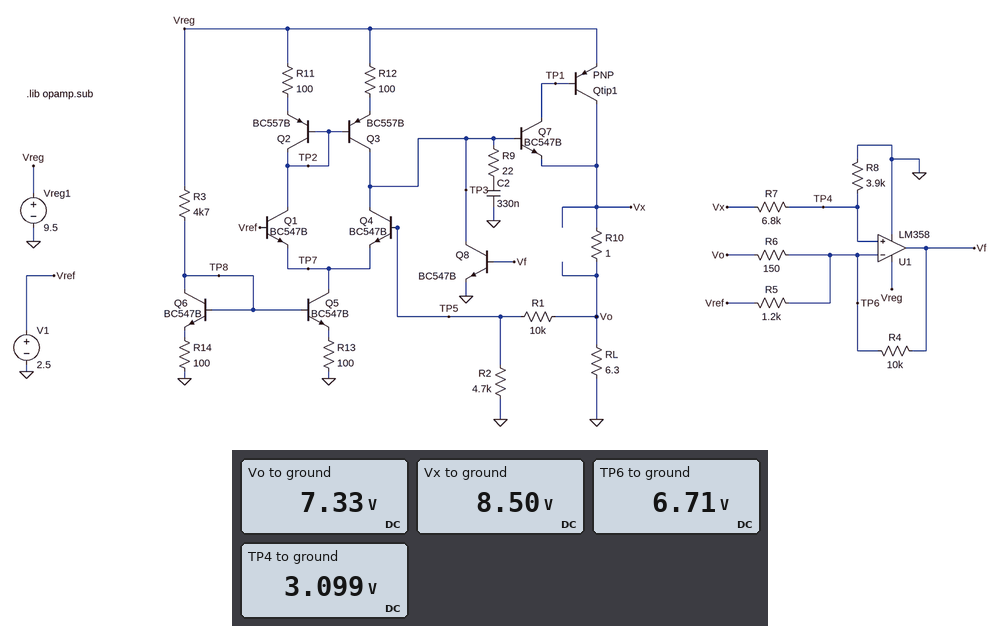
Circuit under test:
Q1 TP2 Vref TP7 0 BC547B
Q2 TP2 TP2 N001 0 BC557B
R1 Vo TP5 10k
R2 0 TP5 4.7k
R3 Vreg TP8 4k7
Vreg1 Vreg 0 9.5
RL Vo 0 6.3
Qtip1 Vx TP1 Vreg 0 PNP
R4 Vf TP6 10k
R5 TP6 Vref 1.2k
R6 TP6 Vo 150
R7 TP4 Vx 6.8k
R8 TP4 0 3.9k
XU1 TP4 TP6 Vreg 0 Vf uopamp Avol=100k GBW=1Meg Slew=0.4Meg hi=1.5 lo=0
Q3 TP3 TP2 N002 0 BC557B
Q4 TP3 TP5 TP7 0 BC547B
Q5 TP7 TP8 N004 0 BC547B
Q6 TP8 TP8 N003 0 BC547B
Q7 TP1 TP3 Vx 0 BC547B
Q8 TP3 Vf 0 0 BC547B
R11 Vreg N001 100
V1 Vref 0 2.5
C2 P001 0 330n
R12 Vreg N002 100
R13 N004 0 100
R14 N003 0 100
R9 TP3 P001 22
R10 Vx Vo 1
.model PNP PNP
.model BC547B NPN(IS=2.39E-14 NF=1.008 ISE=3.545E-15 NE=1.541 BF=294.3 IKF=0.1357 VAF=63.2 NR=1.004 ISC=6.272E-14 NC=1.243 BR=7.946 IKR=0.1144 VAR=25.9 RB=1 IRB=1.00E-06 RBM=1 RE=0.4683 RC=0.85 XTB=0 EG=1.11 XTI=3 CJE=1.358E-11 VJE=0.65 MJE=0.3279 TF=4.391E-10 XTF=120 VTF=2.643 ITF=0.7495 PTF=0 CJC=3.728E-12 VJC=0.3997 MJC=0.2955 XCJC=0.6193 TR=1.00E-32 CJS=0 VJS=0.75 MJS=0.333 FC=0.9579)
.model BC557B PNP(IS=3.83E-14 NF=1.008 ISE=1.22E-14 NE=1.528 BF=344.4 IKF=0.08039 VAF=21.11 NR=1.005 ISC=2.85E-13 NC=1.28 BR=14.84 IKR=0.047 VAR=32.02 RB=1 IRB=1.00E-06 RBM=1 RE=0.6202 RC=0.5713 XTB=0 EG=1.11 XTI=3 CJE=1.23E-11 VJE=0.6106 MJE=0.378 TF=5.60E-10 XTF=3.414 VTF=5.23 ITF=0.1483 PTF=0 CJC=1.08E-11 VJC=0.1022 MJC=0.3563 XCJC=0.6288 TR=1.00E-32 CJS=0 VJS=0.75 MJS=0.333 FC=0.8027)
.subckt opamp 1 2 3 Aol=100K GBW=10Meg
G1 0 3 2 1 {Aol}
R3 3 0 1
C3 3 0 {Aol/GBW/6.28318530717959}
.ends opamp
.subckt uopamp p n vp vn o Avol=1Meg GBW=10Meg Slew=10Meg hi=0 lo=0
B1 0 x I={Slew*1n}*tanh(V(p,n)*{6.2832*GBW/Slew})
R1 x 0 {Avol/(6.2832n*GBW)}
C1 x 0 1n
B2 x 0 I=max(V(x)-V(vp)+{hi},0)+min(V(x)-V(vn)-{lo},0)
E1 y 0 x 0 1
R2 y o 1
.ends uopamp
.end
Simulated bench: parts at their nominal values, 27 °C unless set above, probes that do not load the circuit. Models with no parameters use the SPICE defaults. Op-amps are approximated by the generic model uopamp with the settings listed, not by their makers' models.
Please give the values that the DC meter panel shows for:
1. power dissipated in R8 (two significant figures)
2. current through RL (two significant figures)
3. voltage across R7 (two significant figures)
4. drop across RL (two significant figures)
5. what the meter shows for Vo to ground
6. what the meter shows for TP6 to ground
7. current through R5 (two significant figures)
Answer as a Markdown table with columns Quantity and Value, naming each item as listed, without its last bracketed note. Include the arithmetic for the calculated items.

| Quantity | Value |
|---|---|
| power dissipated in R8 | (3.099 V)^2 / 3.9 kΩ = 2.5 mW |
| current through RL | (7.33 V) / 6.3 Ω = 1.2 A |
| voltage across R7 | 8.5 V - 3.099 V = 5.4 V |
| drop across RL | 7.33 V = 7.3 V |
| what the meter shows for Vo to ground | 7.33 V |
| what the meter shows for TP6 to ground | 6.71 V |
| current through R5 | (6.71 V - 2.5 V) / 1.2 kΩ = 3.5 mA |
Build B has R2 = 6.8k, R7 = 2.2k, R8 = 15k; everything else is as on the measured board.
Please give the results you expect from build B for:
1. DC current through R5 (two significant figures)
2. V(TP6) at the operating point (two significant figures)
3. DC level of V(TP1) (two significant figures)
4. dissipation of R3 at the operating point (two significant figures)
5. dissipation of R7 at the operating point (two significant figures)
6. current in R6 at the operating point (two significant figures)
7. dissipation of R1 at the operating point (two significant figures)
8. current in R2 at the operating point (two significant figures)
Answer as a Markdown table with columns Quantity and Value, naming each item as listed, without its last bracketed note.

| Quantity | Value |
|---|---|
| DC current through R5 | 300 µA |
| V(TP6) at the operating point | 2.1 V |
| DC level of V(TP1) | 8.6 V |
| dissipation of R3 at the operating point | 16 mW |
| dissipation of R7 at the operating point | 45 µW |
| current in R6 at the operating point | 150 µA |
| dissipation of R1 at the operating point | 160 µW |
| current in R2 at the operating point | 130 µA |
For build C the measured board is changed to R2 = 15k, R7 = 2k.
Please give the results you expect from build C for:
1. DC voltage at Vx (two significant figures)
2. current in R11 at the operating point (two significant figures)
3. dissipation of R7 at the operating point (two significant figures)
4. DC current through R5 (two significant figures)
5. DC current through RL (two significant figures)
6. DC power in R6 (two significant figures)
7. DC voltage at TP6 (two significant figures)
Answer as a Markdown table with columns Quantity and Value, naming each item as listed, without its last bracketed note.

| Quantity | Value |
|---|---|
| DC voltage at Vx | 4.9 V |
| current in R11 at the operating point | 910 µA |
| dissipation of R7 at the operating point | 1.4 mW |
| DC current through R5 | 1.2 mA |
| DC current through RL | 670 mA |
| DC power in R6 | 390 µW |
| DC voltage at TP6 | 4.0 V |
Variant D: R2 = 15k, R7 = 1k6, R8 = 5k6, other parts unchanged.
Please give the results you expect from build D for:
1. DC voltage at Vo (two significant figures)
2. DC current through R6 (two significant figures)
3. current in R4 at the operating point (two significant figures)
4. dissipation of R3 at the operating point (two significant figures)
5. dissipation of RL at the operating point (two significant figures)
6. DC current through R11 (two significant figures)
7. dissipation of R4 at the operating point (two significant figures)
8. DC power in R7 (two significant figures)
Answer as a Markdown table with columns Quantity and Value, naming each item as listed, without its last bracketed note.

| Quantity | Value |
|---|---|
| DC voltage at Vo | 4.2 V |
| DC current through R6 | 1.6 mA |
| current in R4 at the operating point | 400 µA |
| dissipation of R3 at the operating point | 16 mW |
| dissipation of RL at the operating point | 2.8 W |
| DC current through R11 | 910 µA |
| dissipation of R4 at the operating point | 1.6 mW |
| DC power in R7 | 730 µW |
